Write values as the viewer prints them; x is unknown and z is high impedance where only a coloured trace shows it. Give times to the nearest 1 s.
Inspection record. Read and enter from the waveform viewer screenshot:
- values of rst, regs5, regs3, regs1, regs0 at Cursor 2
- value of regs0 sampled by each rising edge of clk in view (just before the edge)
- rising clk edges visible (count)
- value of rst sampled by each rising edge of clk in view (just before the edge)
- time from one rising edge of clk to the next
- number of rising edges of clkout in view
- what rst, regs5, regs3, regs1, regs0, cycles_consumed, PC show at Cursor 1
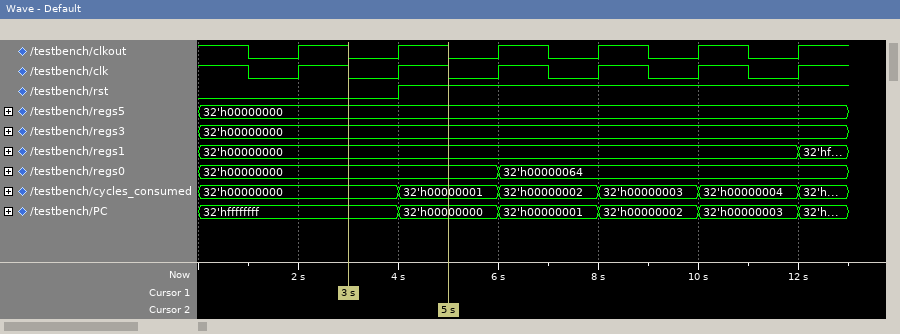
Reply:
rst=1, regs5=32'h00000000, regs3=32'h00000000, regs1=32'h00000000, regs0=32'h00000000
32'h00000000, 32'h00000000, 32'h00000000, 32'h00000064, 32'h00000064, 32'h00000064
6
0 0 1 1 1 1
2 s
6
rst=0, regs5=32'h00000000, regs3=32'h00000000, regs1=32'h00000000, regs0=32'h00000000, cycles_consumed=32'h00000000, PC=32'hffffffff
